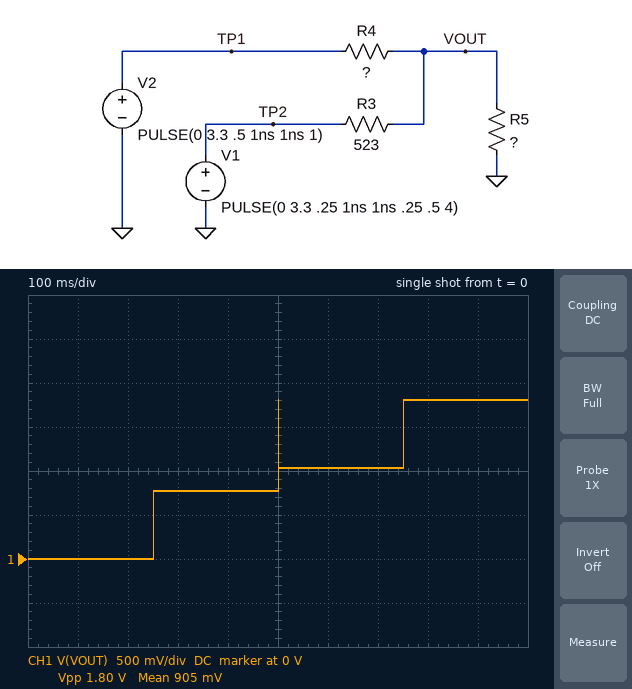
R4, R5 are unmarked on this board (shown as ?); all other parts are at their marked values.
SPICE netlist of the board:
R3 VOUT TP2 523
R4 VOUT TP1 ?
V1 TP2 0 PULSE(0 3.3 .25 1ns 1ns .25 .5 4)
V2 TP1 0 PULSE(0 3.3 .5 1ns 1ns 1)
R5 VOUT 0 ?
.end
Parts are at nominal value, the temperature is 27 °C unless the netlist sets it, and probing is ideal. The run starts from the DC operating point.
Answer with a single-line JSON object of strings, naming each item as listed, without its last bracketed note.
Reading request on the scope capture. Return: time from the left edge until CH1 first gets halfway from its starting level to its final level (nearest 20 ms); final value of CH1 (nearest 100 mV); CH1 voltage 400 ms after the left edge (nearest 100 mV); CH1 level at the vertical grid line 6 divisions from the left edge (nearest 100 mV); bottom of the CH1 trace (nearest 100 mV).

{"time from the left edge until CH1 first gets halfway from its starting level to its final level": "500 ms", "final value of CH1": "1.8 V", "CH1 voltage 400 ms after the left edge": "800 mV", "CH1 level at the vertical grid line 6 divisions from the left edge": "1.0 V", "bottom of the CH1 trace": "0 V"}
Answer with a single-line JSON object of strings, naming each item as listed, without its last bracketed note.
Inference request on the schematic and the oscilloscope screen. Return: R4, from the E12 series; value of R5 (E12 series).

{"R4, from the E12 series": "390 Ω", "value of R5": "270 Ω"}
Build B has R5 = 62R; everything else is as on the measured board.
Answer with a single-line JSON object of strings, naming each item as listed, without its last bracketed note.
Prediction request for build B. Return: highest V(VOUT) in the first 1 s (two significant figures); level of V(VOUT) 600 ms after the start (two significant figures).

{"highest V(VOUT) in the first 1 s": "720 mV", "level of V(VOUT) 600 ms after the start": "410 mV"}
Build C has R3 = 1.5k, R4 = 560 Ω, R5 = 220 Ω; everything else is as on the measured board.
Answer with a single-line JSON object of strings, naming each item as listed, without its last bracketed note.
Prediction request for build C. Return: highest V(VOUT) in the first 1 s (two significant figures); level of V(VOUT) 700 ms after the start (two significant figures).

{"highest V(VOUT) in the first 1 s": "1.2 V", "level of V(VOUT) 700 ms after the start": "840 mV"}
